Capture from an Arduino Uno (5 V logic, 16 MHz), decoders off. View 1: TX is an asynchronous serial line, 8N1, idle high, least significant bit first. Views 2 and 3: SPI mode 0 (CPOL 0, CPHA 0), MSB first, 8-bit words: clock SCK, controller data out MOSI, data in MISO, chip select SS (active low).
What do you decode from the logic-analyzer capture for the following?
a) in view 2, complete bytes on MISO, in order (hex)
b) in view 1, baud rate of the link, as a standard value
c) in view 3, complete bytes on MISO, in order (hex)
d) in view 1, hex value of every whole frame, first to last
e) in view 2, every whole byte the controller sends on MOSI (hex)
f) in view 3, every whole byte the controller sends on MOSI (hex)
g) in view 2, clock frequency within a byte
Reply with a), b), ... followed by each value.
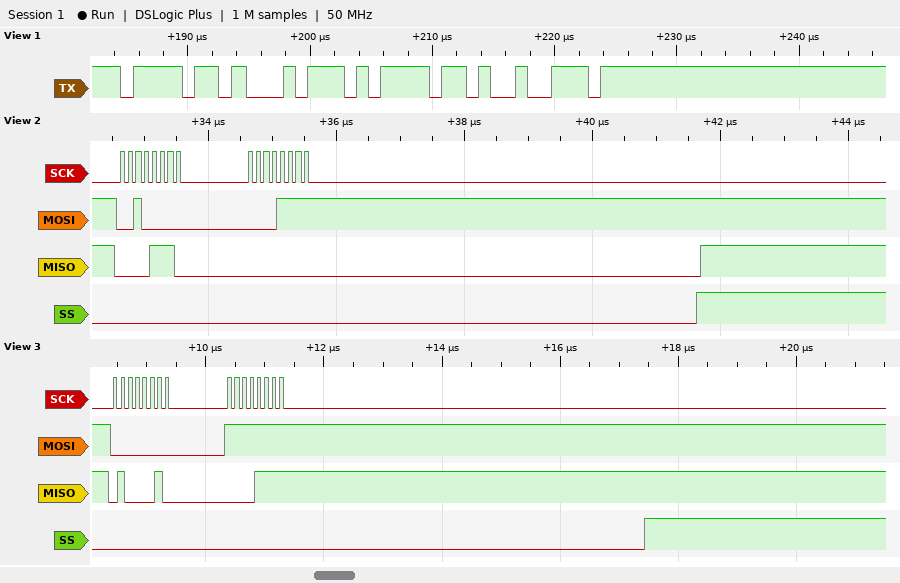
a) 0x0E 0x00
b) 1000000 baud
c) 42 0F
d) 6F 74 6F 72
e) 0x20 0x0F
f) 00 FF
g) 8 MHz
